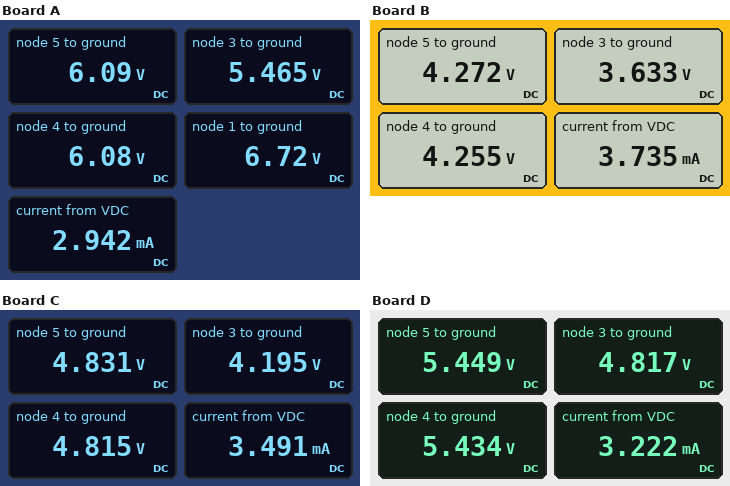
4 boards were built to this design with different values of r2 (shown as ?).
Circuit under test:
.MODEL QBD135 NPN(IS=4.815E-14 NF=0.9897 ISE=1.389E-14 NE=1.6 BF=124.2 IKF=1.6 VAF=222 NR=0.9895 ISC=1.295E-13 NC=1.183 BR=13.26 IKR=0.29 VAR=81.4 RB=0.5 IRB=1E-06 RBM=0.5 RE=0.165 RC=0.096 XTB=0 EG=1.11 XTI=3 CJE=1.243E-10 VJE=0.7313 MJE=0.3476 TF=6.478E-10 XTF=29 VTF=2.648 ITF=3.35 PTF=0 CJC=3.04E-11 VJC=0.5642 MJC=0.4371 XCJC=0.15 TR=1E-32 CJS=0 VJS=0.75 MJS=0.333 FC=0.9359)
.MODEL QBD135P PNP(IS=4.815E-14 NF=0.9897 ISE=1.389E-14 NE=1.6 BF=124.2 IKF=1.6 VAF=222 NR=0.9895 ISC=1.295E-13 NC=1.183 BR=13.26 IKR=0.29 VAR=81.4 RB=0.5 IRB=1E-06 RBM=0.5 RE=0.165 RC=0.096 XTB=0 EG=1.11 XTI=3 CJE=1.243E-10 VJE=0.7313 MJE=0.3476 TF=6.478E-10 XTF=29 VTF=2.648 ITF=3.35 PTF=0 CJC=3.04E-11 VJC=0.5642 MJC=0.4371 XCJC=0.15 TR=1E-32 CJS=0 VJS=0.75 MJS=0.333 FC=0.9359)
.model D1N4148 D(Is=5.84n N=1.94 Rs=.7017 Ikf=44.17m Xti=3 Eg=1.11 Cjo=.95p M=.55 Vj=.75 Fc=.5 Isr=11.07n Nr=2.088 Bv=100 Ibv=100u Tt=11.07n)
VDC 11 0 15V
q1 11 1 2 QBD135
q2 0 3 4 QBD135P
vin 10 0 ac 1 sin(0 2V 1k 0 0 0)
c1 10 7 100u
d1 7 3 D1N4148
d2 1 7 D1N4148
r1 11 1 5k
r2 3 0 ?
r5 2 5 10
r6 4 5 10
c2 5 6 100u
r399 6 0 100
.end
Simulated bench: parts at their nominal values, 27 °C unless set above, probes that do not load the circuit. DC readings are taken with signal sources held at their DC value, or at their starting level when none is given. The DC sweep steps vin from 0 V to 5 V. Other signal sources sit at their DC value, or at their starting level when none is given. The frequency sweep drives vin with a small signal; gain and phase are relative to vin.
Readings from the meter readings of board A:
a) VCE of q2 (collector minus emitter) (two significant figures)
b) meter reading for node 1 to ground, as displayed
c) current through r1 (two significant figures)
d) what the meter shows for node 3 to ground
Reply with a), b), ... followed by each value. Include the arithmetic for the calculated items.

a) 0 V - 6.08 V = -6.1 V
b) 6.72 V
c) (15 V - 6.72 V) / 5 kΩ = 1.7 mA
d) 5.465 V
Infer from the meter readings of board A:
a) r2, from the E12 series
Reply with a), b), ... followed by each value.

a) 3.3 kΩ
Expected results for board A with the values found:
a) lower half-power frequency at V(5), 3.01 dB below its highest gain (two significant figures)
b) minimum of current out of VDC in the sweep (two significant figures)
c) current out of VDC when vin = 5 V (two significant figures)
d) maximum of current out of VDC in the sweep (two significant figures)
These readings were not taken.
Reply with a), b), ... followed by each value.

a) 750 mHz
b) 2.9 mA
c) 2.9 mA
d) 2.9 mA
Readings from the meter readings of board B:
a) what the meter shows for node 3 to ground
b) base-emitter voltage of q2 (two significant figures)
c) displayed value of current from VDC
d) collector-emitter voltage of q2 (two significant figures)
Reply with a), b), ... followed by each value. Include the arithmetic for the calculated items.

a) 3.633 V
b) 3.633 V - 4.255 V = -620 mV
c) 3.735 mA
d) 0 V - 4.255 V = -4.3 V
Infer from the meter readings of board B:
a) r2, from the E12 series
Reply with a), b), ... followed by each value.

a) 1.8 kΩ
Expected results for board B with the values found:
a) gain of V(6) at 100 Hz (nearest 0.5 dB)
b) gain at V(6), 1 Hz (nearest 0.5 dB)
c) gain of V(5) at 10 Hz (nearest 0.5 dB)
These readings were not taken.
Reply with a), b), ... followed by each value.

a) -1.0 dB
b) -28.0 dB
c) -0.5 dB
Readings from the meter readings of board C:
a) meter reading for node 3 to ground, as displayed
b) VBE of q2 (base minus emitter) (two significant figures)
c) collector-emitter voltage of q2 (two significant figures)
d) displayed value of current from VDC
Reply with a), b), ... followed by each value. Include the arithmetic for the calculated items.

a) 4.195 V
b) 4.195 V - 4.815 V = -620 mV
c) 0 V - 4.815 V = -4.8 V
d) 3.491 mA
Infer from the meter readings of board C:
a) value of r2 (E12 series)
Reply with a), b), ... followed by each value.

a) 2.2 kΩ
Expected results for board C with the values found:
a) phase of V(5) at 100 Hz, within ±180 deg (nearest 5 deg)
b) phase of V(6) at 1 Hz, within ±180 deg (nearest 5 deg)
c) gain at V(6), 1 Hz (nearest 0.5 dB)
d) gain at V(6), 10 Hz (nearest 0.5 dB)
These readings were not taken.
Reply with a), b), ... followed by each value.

a) 0 deg
b) 130 deg
c) -27.5 dB
d) -6.0 dB
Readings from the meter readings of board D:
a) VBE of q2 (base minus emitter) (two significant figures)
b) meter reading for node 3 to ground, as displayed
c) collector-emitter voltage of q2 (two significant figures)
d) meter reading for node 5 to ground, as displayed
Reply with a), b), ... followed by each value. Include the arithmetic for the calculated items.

a) 4.817 V - 5.434 V = -620 mV
b) 4.817 V
c) 0 V - 5.434 V = -5.4 V
d) 5.449 V
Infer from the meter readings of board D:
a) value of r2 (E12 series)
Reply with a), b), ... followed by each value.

a) 2.7 kΩ
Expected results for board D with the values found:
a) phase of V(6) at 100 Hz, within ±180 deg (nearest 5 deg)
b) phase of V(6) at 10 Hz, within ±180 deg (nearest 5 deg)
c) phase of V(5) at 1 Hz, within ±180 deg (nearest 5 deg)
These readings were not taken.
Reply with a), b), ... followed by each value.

a) 10 deg
b) 60 deg
c) 40 deg
